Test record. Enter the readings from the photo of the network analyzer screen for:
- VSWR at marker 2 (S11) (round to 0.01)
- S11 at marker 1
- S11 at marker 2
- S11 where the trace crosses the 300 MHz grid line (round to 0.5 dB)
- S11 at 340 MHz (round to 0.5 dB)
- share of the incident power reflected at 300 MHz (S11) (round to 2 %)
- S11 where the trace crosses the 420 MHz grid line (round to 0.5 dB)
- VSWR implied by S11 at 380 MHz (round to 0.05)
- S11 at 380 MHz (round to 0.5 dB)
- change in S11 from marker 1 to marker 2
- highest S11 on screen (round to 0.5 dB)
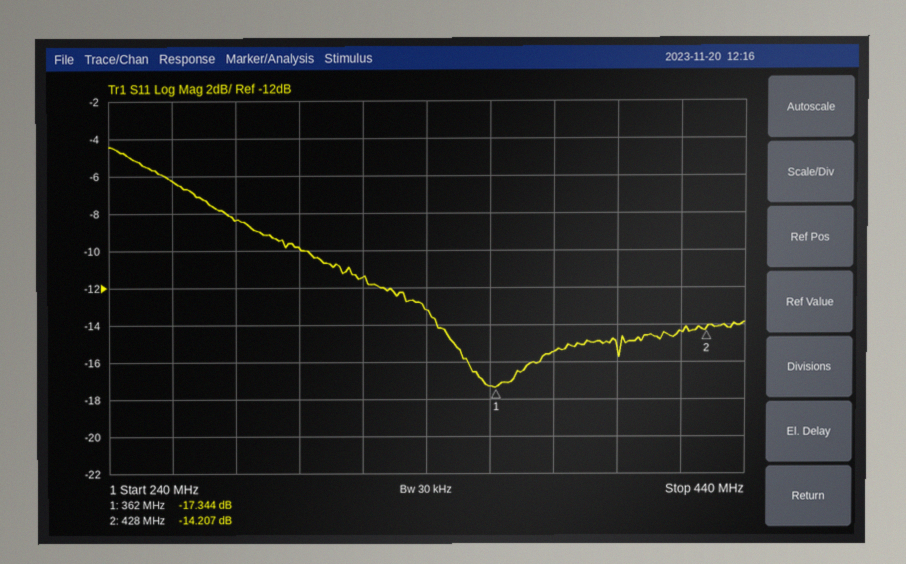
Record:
1.48
-17.344 dB
-14.207 dB
-10.0 dB
-13.0 dB
10 %
-14.5 dB
1.40
-15.5 dB
3.137 dB
-4.5 dB
